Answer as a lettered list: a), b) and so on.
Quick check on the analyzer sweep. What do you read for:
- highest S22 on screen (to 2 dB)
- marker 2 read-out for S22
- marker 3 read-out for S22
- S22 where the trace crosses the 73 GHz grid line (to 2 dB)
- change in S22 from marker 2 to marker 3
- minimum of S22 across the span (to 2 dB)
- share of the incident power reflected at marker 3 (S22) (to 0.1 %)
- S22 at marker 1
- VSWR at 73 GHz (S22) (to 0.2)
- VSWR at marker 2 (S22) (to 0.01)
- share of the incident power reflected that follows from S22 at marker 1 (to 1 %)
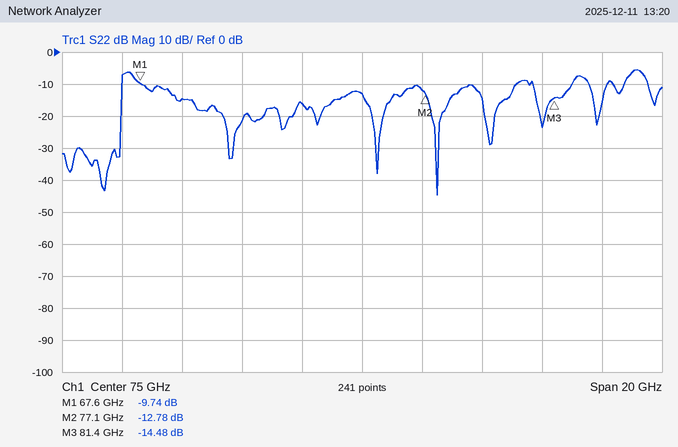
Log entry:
a) -6 dB
b) -12.78 dB
c) -14.48 dB
d) -16 dB
e) -1.70 dB
f) -44 dB
g) 3.6 %
h) -9.74 dB
i) 1.4
j) 1.60
k) 11 %
